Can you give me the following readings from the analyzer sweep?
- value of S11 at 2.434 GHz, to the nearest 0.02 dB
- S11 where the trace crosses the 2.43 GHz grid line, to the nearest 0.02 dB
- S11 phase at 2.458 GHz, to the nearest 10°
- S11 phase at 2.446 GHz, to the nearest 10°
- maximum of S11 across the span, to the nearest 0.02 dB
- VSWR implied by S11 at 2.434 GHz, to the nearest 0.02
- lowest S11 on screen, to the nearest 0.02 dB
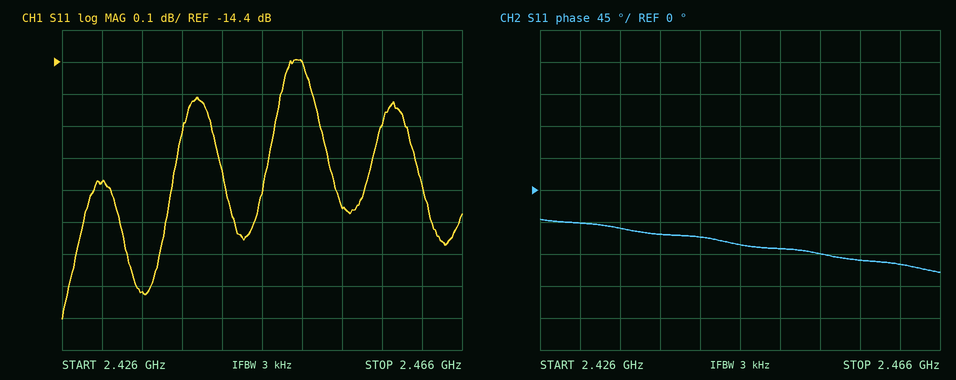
-15.12 dB
-14.78 dB
-100°
-80°
-14.40 dB
1.42
-15.20 dB
